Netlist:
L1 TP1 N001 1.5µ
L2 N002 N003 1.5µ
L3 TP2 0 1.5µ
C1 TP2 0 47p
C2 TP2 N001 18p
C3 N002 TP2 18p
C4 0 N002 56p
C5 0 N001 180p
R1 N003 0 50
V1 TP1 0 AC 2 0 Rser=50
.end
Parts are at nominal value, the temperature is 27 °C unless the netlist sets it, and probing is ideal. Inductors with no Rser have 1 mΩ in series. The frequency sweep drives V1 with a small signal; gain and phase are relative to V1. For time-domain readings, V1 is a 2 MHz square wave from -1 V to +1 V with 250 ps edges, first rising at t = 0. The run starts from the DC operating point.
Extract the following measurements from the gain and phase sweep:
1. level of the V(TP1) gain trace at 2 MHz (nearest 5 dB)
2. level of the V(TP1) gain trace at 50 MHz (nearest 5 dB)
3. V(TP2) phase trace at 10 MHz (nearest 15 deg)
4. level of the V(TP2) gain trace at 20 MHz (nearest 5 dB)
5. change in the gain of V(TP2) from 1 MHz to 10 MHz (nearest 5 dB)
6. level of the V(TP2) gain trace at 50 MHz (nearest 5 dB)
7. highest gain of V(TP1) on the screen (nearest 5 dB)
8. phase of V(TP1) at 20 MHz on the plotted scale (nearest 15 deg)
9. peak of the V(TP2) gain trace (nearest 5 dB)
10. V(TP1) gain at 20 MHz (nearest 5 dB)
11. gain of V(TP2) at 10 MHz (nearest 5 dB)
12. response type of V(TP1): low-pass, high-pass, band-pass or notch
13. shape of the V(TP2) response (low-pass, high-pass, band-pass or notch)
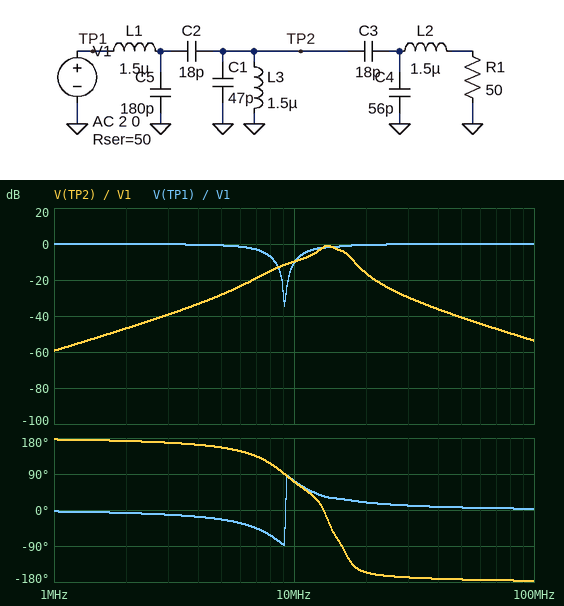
0 dB
0 dB
75 deg
-15 dB
50 dB
-40 dB
0 dB
15 deg
0 dB
0 dB
-10 dB
notch
band-pass
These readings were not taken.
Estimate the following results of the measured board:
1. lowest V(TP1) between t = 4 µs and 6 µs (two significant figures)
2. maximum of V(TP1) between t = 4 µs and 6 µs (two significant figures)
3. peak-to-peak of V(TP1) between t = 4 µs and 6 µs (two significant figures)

-1.3 V
1.3 V
2.6 V
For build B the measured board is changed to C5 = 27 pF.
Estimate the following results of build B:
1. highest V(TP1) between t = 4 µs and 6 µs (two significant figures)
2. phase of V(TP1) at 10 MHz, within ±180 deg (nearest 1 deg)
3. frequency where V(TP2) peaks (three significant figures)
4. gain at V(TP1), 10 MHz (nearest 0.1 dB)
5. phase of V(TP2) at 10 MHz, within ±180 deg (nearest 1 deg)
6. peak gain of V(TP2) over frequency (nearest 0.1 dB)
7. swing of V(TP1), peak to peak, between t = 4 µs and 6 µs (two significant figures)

1.2 V
-12 deg
13.5 MHz
-0.2 dB
166 deg
7.0 dB
2.4 V
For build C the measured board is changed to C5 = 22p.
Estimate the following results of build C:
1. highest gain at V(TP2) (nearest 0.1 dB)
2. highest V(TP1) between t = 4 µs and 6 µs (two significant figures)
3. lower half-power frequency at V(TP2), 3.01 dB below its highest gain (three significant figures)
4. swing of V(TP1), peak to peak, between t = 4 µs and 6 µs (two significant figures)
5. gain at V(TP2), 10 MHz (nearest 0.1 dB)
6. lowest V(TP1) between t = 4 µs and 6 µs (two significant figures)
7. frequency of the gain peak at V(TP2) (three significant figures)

6.7 dB
1.2 V
12.7 MHz
2.4 V
-10.9 dB
-1.2 V
13.5 MHz
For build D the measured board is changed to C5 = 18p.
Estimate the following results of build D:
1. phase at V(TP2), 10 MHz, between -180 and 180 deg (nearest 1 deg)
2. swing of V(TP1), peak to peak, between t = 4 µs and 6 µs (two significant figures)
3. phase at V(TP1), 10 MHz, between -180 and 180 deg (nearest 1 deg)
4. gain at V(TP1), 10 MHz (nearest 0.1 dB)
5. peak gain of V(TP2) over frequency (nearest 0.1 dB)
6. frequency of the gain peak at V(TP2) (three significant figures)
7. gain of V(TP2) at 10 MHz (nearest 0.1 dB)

169 deg
2.4 V
-9 deg
-0.1 dB
6.4 dB
13.5 MHz
-11.1 dB
